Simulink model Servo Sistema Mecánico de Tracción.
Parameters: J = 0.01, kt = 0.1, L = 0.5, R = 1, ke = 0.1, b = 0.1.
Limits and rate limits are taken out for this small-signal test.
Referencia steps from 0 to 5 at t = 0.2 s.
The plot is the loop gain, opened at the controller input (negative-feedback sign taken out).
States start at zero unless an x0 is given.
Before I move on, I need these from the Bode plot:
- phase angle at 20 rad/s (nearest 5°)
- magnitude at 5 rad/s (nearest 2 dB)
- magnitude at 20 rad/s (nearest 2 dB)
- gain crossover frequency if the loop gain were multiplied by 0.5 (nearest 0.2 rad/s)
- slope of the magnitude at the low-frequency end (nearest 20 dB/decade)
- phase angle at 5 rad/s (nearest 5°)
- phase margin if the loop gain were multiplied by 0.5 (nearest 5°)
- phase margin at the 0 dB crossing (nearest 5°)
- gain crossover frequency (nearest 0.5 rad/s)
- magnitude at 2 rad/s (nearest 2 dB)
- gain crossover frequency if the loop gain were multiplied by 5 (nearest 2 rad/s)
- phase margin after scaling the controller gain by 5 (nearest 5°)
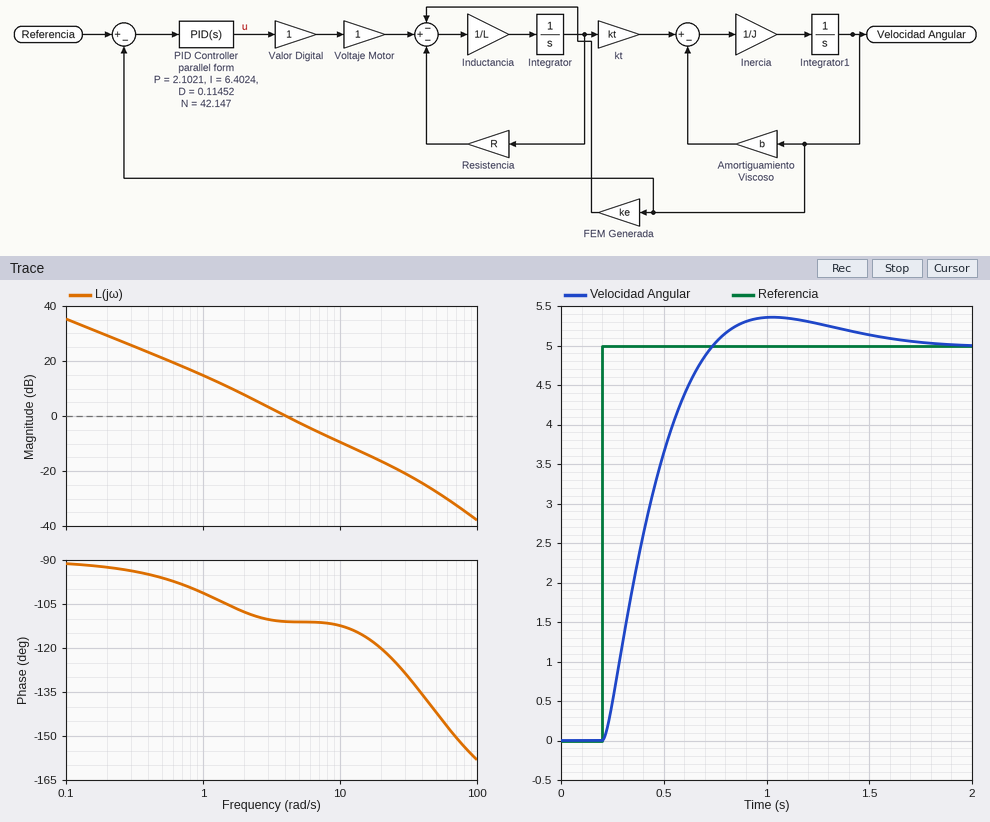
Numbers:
-120°
-2 dB
-16 dB
2.4 rad/s
-20 dB/decade
-110°
70°
70°
4.0 rad/s
8 dB
16 rad/s
65°
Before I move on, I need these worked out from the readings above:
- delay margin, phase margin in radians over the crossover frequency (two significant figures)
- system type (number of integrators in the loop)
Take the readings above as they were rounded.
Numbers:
0.31 s
1
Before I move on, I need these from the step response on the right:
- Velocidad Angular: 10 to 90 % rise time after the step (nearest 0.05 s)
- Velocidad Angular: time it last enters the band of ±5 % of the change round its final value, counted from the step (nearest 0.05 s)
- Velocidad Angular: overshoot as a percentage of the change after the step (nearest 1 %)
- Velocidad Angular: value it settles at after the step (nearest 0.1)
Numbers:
0.35 s
1.10 s
7 %
5.0
